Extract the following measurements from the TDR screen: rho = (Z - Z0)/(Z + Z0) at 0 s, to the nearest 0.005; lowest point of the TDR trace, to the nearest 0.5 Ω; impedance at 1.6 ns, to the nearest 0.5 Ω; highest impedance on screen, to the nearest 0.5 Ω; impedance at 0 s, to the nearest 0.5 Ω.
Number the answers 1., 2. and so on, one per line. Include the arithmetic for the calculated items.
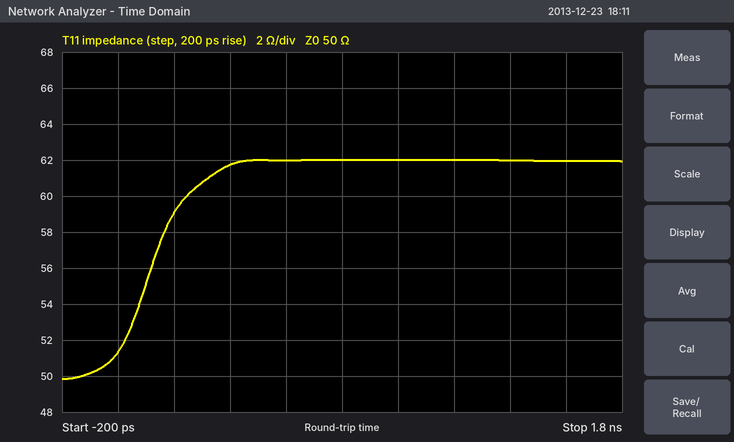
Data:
1. (51.5 − 50)/(51.5 + 50) ≈ +0.015
2. 50.0 Ω
3. 62.0 Ω
4. 62.0 Ω
5. 51.5 Ω
